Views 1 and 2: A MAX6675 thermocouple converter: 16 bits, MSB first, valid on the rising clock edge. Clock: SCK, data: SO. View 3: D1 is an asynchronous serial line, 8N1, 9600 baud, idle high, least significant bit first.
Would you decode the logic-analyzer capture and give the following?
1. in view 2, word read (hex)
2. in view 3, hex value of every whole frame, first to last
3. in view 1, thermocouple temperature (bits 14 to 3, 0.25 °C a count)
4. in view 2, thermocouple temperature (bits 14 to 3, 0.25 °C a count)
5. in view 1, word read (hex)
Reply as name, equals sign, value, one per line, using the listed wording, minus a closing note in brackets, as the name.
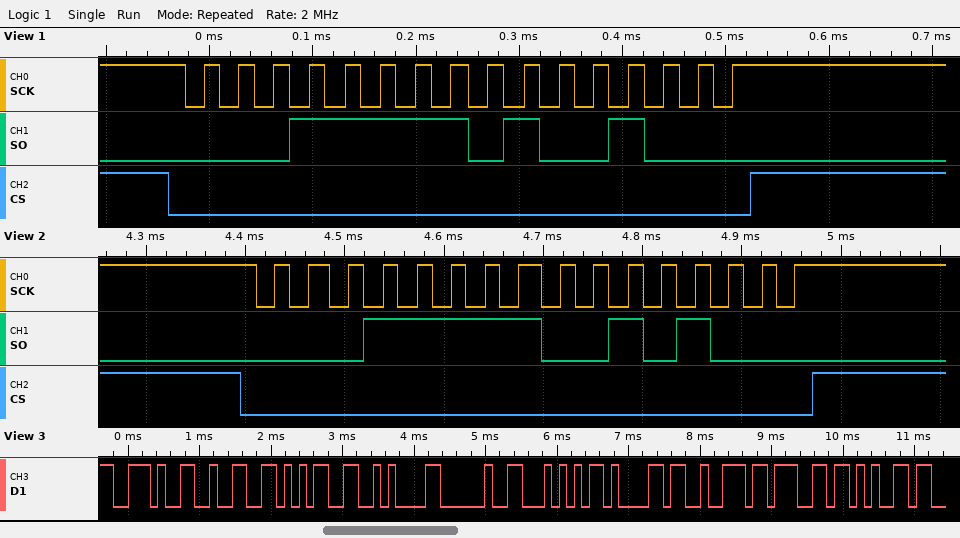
in view 2, word read = 0x1F28
in view 3, hex value of every whole frame, first to last = 2E 32 35 0A 20 54 61 72 67 65
in view 1, thermocouple temperature = 250.25 °C
in view 2, thermocouple temperature = 249.25 °C
in view 1, word read = 0x1F48
